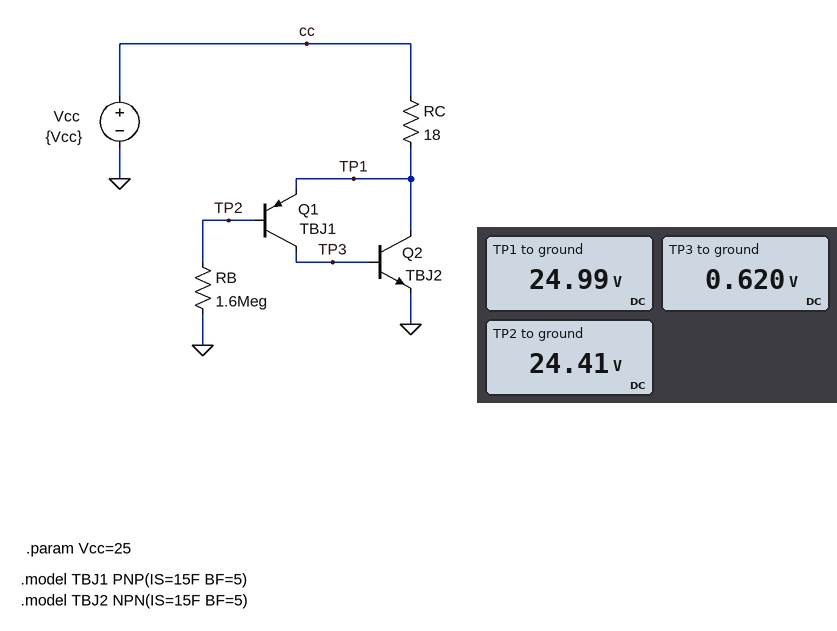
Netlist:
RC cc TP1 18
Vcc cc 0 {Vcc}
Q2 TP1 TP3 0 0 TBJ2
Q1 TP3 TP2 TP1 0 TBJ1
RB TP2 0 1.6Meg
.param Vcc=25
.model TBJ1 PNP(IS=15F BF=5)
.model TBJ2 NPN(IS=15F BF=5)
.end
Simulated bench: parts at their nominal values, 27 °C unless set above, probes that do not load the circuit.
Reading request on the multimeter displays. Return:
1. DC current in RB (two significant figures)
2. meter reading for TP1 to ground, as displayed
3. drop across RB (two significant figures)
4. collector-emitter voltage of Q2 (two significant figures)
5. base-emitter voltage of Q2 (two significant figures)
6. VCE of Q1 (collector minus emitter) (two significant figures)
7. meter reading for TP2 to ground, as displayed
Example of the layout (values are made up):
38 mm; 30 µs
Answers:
15 µA; 24.99 V; 24 V; 25 V; 620 mV; -24 V; 24.41 V
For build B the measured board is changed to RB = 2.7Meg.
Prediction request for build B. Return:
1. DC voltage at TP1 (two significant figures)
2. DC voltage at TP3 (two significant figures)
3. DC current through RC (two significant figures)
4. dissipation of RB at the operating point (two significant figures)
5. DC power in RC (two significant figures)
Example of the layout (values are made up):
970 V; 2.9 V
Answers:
25 V; 610 mV; 280 µA; 220 µW; 1.4 µW
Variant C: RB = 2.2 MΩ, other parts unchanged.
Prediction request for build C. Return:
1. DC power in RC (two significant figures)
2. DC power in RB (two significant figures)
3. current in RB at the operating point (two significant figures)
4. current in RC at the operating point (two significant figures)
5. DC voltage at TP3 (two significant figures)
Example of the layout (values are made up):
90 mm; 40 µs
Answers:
2.1 µW; 270 µW; 11 µA; 340 µA; 610 mV
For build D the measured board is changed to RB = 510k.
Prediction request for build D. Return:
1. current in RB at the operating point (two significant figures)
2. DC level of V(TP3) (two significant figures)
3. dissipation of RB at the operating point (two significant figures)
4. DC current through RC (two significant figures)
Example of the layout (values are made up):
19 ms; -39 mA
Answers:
48 µA; 650 mV; 1.2 mW; 1.5 mA
